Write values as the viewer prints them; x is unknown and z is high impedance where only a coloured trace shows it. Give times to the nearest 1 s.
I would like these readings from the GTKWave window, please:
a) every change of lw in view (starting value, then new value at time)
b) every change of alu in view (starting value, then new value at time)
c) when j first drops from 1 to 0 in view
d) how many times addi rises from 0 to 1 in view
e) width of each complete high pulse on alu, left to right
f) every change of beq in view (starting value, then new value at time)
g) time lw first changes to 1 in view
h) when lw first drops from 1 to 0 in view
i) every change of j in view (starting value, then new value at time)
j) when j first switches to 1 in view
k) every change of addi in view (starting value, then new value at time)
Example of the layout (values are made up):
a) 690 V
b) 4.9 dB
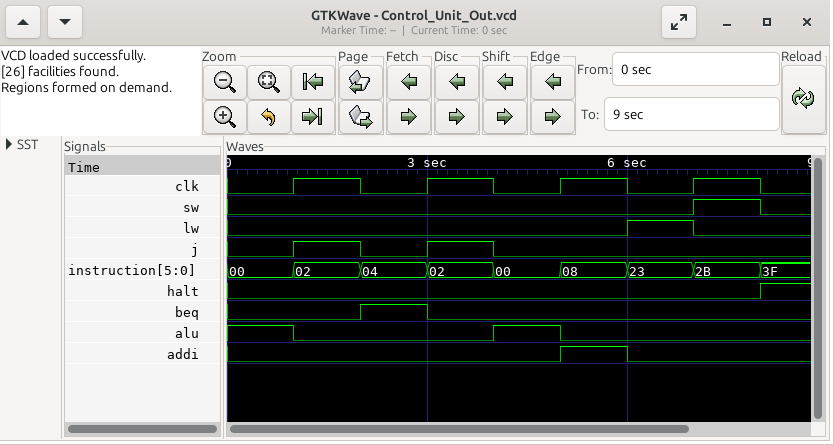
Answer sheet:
a) 0, 1 at 6 s, 0 at 7 s
b) 1, 0 at 1 s, 1 at 4 s, 0 at 5 s
c) 2 s
d) 1
e) 1 s
f) 0, 1 at 2 s, 0 at 3 s
g) 6 s
h) 7 s
i) 0, 1 at 1 s, 0 at 2 s, 1 at 3 s, 0 at 4 s
j) 1 s
k) 0, 1 at 5 s, 0 at 6 s
